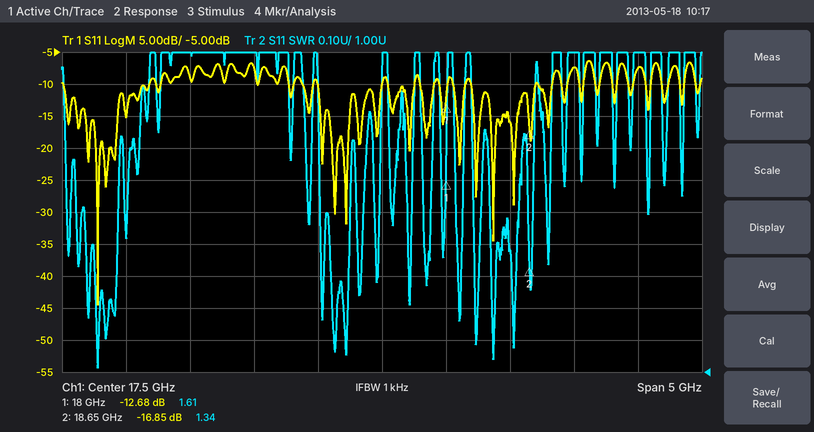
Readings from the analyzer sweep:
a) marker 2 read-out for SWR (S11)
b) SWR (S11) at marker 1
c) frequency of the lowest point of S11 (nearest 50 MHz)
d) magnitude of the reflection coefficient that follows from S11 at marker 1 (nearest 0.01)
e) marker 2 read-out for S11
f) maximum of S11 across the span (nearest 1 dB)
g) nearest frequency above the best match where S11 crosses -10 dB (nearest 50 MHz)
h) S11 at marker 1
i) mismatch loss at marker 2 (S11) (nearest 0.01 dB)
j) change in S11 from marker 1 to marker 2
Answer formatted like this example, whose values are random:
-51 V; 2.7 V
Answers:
1.34; 1.61; 15.30 GHz; 0.23; -16.85 dB; -6 dB; 15.70 GHz; -12.68 dB; 0.09 dB; -4.17 dB
